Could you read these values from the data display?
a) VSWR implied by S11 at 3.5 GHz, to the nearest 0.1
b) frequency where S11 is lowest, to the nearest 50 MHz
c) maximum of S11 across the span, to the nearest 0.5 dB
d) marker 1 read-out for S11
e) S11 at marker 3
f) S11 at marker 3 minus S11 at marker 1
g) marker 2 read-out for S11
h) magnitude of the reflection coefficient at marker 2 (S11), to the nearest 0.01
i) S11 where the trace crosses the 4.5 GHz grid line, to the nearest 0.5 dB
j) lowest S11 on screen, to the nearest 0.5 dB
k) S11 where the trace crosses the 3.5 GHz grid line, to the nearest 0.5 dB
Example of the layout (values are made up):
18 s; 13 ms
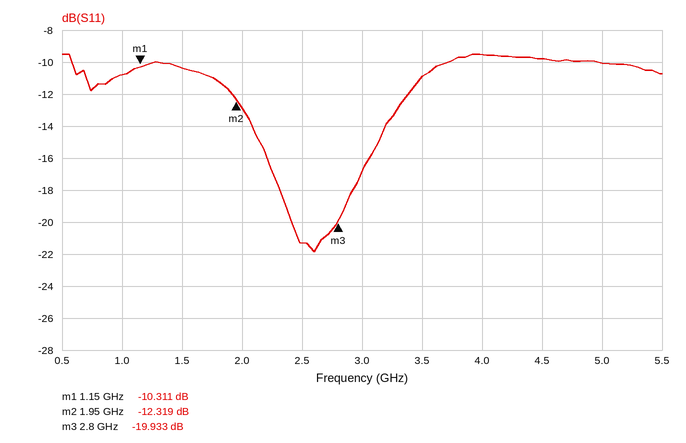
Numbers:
1.8; 2.60 GHz; -9.5 dB; -10.311 dB; -19.933 dB; -9.622 dB; -12.319 dB; 0.24; -10.0 dB; -22.0 dB; -11.0 dB
